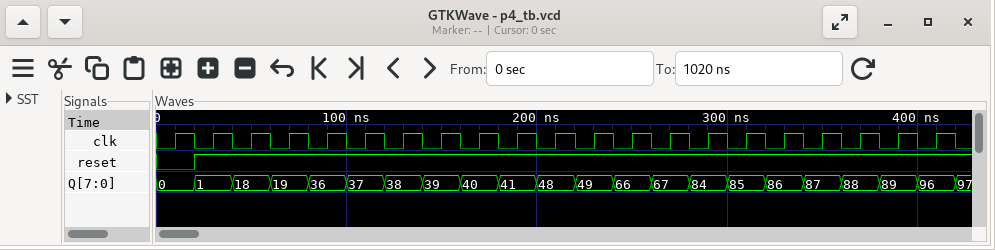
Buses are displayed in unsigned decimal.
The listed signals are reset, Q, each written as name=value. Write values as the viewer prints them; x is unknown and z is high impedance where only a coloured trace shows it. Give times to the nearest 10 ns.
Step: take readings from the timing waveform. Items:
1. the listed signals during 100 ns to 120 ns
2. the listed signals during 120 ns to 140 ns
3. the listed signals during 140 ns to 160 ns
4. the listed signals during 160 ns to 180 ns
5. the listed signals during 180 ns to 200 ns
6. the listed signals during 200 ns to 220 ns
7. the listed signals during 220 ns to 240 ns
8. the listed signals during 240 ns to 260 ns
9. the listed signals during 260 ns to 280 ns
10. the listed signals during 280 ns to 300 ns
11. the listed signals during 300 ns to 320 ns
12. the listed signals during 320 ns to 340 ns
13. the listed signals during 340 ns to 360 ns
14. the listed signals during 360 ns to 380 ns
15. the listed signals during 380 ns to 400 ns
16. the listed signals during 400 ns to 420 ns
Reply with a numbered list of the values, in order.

1. reset=1, Q=37
2. reset=1, Q=38
3. reset=1, Q=39
4. reset=1, Q=40
5. reset=1, Q=41
6. reset=1, Q=48
7. reset=1, Q=49
8. reset=1, Q=66
9. reset=1, Q=67
10. reset=1, Q=84
11. reset=1, Q=85
12. reset=1, Q=86
13. reset=1, Q=87
14. reset=1, Q=88
15. reset=1, Q=89
16. reset=1, Q=96
